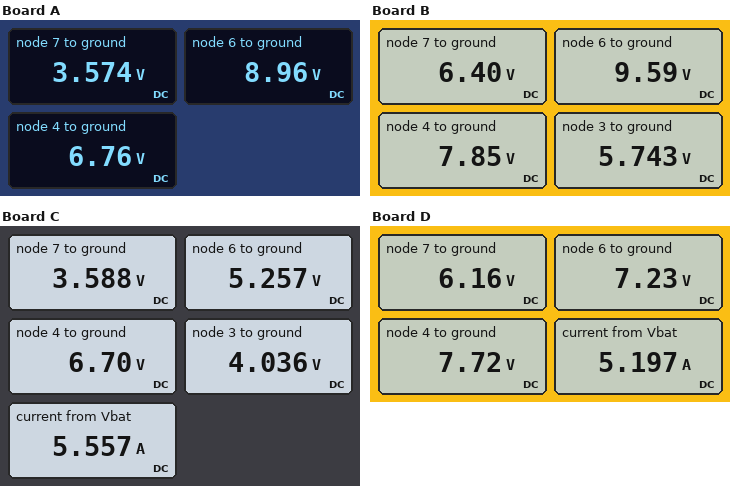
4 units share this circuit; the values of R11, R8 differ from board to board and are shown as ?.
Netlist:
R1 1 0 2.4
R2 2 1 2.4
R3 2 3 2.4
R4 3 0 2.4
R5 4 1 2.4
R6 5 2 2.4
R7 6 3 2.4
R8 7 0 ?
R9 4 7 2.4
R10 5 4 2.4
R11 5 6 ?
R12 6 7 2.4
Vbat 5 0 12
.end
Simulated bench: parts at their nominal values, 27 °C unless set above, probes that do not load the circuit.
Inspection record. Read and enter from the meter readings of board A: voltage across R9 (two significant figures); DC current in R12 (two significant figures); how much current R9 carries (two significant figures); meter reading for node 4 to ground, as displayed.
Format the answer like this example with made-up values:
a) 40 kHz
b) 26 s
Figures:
a) 3.2 V
b) 2.2 A
c) 1.3 A
d) 6.76 V
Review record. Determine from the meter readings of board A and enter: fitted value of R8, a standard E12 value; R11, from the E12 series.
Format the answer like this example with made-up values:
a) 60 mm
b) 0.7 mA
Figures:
a) 1 Ω
b) 0.82 Ω
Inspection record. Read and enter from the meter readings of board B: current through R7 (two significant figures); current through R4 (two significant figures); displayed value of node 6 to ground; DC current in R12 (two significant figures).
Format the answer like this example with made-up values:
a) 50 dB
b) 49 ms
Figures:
a) 1.6 A
b) 2.4 A
c) 9.59 V
d) 1.3 A
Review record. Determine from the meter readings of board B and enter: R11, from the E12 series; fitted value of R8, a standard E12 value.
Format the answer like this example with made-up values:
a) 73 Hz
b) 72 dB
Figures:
a) 0.82 Ω
b) 3.3 Ω
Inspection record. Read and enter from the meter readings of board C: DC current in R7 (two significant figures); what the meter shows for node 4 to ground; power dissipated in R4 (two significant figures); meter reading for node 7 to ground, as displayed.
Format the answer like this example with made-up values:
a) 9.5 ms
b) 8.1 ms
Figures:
a) 510 mA
b) 6.70 V
c) 6.8 W
d) 3.588 V
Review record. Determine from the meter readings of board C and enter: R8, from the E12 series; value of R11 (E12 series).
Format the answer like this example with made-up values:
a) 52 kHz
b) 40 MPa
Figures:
a) 1.8 Ω
b) 5.6 Ω
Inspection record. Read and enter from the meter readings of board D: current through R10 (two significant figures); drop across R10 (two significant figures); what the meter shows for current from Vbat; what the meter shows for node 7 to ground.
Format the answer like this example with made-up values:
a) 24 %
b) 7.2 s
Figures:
a) 1.8 A
b) 4.3 V
c) 5.197 A
d) 6.16 V
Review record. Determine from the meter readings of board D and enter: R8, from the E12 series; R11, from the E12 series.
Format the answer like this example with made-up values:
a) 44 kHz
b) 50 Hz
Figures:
a) 5.6 Ω
b) 3.3 Ω
